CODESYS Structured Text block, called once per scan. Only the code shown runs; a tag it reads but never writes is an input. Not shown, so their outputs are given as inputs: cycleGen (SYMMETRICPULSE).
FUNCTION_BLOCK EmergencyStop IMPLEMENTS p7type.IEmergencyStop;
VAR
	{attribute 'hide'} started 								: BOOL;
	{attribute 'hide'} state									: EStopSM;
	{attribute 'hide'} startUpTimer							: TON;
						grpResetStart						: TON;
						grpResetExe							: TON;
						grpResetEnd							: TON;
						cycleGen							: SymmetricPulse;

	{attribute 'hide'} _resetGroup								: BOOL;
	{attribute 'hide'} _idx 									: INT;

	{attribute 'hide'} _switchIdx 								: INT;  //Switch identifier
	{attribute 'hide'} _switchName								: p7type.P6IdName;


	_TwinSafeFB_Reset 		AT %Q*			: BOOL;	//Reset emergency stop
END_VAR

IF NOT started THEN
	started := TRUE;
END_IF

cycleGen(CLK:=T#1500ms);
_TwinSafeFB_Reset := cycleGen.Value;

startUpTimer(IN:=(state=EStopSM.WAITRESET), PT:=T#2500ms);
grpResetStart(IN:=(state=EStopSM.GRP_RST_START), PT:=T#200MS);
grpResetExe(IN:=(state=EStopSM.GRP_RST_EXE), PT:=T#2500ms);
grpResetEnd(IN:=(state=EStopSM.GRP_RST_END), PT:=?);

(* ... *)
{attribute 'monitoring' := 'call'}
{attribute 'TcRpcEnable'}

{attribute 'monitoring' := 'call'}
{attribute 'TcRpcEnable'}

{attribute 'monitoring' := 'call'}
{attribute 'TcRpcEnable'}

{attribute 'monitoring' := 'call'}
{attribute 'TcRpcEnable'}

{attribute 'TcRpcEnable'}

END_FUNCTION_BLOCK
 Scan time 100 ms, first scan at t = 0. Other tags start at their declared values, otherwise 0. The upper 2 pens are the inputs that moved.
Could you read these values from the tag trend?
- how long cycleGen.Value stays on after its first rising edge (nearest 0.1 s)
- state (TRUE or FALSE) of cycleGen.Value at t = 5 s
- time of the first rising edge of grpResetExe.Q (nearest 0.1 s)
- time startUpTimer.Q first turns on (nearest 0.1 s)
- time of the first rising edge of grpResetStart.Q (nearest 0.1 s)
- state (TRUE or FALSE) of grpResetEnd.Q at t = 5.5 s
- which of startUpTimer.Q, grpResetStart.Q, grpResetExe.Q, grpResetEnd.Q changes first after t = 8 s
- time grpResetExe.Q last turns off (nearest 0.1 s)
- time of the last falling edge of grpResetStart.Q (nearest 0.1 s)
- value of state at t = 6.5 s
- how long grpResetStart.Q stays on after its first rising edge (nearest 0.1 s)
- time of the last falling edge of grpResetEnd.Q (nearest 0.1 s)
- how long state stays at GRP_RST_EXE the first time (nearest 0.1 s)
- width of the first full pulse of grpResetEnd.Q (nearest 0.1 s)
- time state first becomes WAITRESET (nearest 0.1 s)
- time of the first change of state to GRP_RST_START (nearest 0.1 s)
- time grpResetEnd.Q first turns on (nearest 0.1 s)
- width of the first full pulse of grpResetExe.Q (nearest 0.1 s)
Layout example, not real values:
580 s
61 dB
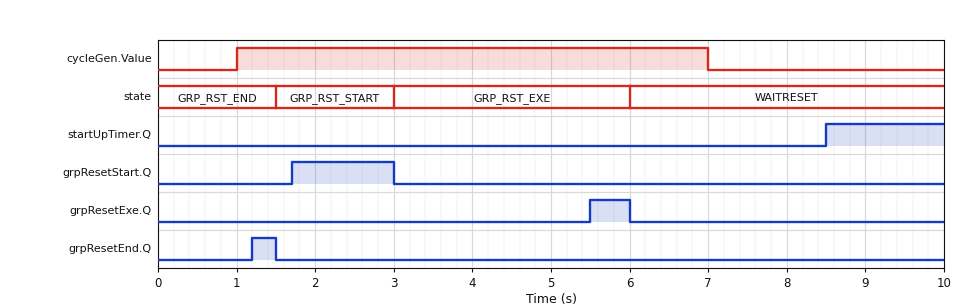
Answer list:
6.0 s
TRUE
5.5 s
8.5 s
1.7 s
FALSE
startUpTimer.Q
6.0 s
3.0 s
WAITRESET
1.3 s
1.5 s
3.0 s
0.3 s
6.0 s
1.5 s
1.2 s
0.5 s
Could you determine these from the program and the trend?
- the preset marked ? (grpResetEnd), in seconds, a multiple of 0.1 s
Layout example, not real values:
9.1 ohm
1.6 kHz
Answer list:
1.2 s
